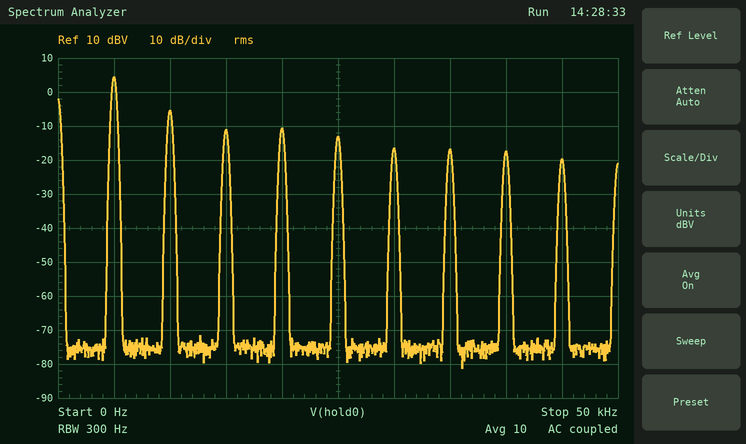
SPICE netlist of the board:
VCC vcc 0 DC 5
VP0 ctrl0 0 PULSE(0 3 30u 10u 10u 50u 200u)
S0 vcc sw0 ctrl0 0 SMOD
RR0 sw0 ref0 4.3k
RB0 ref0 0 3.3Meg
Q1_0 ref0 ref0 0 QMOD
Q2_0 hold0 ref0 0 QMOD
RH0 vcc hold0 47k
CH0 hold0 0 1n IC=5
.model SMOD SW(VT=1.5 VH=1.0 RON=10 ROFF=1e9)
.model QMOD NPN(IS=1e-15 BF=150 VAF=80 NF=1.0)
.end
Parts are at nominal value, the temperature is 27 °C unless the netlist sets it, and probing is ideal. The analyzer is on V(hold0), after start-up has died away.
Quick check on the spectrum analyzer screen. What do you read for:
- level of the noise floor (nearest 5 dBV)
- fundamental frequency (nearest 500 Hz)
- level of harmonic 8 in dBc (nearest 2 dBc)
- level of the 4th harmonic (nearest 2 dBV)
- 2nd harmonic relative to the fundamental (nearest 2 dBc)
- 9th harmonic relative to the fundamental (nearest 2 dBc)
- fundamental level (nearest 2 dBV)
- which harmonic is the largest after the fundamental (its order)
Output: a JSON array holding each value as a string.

["-75 dBV", "5.0 kHz", "-22 dBc", "-10 dBV", "-10 dBc", "-24 dBc", "4 dBV", "2"]
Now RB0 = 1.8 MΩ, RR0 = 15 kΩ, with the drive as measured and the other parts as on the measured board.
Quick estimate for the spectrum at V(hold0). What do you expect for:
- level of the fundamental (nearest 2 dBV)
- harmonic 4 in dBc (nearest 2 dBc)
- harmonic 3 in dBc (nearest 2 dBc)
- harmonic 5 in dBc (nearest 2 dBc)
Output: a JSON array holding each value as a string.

["4 dBV", "-18 dBc", "-18 dBc", "-20 dBc"]
